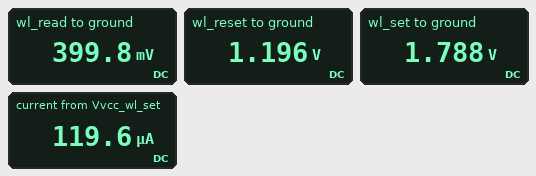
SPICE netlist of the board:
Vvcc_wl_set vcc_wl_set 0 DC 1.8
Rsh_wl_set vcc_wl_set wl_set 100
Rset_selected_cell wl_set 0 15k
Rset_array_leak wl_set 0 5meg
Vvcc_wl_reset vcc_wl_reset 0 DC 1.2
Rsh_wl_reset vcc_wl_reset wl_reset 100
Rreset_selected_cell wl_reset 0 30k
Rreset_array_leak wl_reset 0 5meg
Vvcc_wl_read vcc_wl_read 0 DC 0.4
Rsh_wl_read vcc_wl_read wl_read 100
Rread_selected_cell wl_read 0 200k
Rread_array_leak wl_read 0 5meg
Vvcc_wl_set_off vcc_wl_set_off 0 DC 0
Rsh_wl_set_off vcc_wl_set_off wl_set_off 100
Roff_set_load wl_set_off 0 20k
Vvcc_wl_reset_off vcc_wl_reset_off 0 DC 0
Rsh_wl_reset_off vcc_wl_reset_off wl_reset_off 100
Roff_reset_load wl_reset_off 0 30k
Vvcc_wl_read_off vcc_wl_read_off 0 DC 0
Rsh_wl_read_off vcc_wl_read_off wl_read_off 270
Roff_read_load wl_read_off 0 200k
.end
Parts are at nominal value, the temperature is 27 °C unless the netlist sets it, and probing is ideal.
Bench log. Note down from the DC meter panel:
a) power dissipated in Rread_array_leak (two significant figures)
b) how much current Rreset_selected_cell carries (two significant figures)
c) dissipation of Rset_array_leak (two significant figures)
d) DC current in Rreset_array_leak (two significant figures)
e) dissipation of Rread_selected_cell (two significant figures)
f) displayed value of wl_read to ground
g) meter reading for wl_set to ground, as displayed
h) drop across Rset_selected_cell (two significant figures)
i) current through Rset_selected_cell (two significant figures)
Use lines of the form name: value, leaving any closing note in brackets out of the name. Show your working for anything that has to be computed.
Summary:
power dissipated in Rread_array_leak: (399.8 mV)^2 / 5 MΩ = 32 nW
how much current Rreset_selected_cell carries: (1.196 V) / 30 kΩ = 40 µA
dissipation of Rset_array_leak: (1.788 V)^2 / 5 MΩ = 640 nW
DC current in Rreset_array_leak: (1.196 V) / 5 MΩ = 240 nA
dissipation of Rread_selected_cell: (399.8 mV)^2 / 200 kΩ = 800 nW
displayed value of wl_read to ground: 399.8 mV
meter reading for wl_set to ground, as displayed: 1.788 V
drop across Rset_selected_cell: 1.788 V = 1.8 V
current through Rset_selected_cell: (1.788 V) / 15 kΩ = 120 µA
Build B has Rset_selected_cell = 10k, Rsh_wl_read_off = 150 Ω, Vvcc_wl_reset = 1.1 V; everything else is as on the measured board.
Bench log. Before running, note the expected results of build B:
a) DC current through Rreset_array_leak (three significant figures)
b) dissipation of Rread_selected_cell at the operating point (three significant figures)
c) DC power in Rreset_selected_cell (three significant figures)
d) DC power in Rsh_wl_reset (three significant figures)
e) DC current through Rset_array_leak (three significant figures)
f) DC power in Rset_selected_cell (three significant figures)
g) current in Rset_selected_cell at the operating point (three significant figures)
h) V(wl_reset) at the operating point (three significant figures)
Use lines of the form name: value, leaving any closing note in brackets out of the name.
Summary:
DC current through Rreset_array_leak: 219 nA
dissipation of Rread_selected_cell at the operating point: 799 nW
DC power in Rreset_selected_cell: 40.1 µW
DC power in Rsh_wl_reset: 135 nW
DC current through Rset_array_leak: 356 nA
DC power in Rset_selected_cell: 318 µW
current in Rset_selected_cell at the operating point: 178 µA
V(wl_reset) at the operating point: 1.10 V
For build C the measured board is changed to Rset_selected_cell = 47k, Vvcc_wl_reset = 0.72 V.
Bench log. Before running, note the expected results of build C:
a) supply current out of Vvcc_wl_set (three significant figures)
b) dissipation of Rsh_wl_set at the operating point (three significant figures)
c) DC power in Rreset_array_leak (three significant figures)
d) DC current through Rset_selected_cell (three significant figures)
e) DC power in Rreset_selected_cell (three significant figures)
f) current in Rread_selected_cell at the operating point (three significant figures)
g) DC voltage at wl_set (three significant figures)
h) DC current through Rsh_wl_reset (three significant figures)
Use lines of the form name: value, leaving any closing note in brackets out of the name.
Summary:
supply current out of Vvcc_wl_set: 38.6 µA
dissipation of Rsh_wl_set at the operating point: 149 nW
DC power in Rreset_array_leak: 103 nW
DC current through Rset_selected_cell: 38.2 µA
DC power in Rreset_selected_cell: 17.2 µW
current in Rread_selected_cell at the operating point: 2.00 µA
DC voltage at wl_set: 1.80 V
DC current through Rsh_wl_reset: 24.1 µA
